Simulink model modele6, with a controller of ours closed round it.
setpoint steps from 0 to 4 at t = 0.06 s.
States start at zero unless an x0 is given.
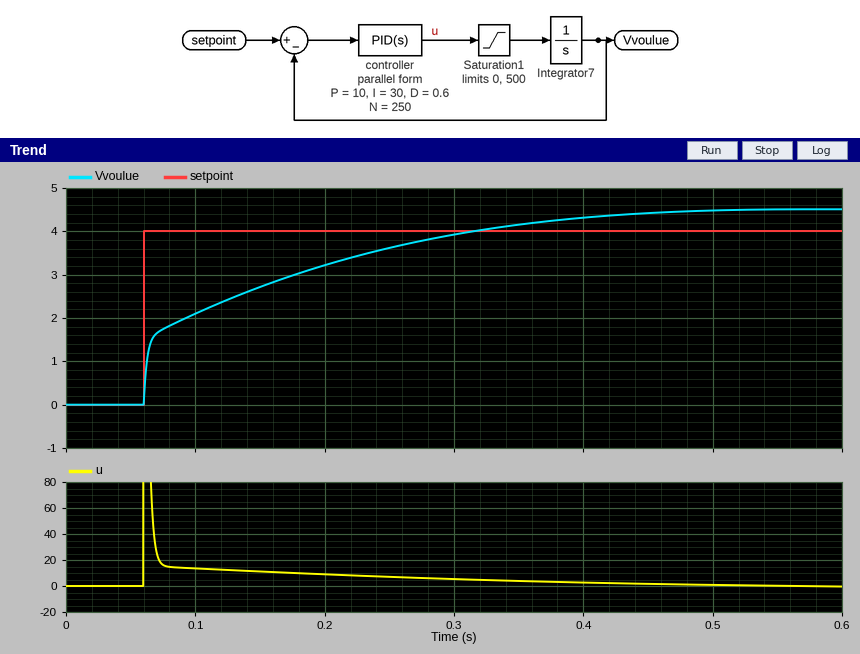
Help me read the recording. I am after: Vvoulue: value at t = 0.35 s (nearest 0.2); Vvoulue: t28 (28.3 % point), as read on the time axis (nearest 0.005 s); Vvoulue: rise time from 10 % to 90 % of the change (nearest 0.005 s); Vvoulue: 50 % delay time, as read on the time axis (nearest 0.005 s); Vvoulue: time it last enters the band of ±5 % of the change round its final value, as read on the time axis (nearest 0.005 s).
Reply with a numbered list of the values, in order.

1. 4.2
2. 0.065 s
3. 0.265 s
4. 0.110 s
5. 0.390 s
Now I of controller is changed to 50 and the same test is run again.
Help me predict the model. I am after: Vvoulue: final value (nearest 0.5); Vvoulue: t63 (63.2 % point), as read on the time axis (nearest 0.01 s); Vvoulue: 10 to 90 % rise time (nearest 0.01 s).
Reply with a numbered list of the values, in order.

1. 4.5
2. 0.16 s
3. 0.24 s
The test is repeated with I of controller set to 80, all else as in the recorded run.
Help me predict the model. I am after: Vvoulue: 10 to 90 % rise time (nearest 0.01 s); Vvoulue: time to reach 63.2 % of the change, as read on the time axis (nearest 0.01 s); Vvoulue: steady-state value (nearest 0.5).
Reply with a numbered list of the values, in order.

1. 0.21 s
2. 0.16 s
3. 5.0
